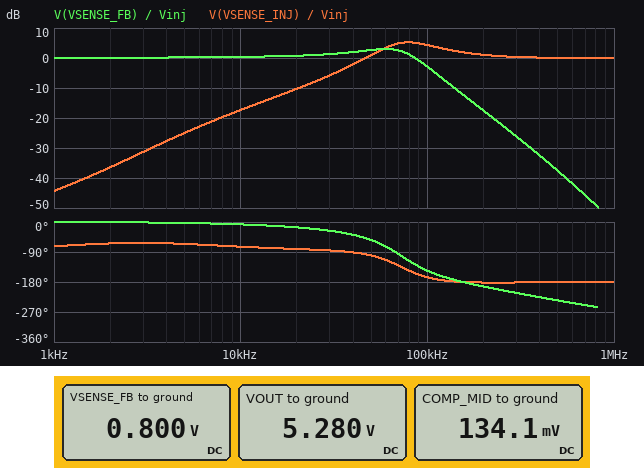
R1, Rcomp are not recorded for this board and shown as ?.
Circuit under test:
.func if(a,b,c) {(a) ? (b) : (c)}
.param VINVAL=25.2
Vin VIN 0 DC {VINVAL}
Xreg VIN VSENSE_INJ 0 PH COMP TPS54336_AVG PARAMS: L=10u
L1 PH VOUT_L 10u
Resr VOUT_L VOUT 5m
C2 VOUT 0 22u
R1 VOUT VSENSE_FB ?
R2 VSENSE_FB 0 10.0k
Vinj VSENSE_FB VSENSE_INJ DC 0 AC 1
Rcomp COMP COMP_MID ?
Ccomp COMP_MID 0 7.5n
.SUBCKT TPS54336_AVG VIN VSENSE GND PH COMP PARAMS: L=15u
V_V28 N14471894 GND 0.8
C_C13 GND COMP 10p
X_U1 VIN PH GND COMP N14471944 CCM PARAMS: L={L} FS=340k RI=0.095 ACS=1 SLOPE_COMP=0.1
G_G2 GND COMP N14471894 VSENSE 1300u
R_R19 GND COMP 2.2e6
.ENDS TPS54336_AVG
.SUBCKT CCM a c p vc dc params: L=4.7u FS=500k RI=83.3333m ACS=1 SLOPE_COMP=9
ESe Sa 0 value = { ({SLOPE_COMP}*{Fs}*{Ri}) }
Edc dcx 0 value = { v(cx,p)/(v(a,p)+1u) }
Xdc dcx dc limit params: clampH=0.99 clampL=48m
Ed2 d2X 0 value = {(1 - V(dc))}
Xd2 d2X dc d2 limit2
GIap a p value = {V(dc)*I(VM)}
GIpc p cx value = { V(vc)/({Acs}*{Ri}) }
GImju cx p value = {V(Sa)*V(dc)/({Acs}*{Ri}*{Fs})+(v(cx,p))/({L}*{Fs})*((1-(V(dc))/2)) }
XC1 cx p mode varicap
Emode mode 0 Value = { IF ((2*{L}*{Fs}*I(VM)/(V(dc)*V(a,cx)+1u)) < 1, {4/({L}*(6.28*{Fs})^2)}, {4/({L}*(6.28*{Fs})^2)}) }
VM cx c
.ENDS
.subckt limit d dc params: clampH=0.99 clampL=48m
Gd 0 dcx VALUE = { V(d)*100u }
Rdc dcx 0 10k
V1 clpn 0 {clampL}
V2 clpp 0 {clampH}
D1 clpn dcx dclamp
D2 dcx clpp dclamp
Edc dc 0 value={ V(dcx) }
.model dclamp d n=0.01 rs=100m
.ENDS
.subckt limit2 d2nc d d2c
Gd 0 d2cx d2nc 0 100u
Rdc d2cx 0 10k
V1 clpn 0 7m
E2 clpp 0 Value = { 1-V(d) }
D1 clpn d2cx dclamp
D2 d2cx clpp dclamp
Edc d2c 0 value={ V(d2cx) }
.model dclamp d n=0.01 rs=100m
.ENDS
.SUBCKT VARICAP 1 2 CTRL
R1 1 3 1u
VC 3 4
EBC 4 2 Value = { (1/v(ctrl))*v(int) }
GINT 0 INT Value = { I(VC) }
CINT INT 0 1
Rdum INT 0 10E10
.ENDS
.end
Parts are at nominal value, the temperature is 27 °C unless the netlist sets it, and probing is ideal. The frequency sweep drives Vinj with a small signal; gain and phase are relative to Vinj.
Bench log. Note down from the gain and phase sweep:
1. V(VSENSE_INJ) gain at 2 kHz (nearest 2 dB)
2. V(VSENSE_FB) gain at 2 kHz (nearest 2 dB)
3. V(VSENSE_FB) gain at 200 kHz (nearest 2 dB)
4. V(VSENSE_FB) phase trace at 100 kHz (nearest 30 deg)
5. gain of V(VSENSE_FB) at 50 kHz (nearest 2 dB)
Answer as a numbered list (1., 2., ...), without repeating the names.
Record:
1. -36 dB
2. 0 dB
3. -18 dB
4. -150 deg
5. 2 dB
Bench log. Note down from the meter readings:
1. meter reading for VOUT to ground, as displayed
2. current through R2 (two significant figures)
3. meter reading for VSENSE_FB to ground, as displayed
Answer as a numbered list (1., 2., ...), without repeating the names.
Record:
1. 5.280 V
2. 80 µA
3. 0.800 V
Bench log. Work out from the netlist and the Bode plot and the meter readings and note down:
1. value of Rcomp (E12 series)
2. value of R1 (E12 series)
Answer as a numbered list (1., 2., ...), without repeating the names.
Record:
1. 4.7 kΩ
2. 56 kΩ
